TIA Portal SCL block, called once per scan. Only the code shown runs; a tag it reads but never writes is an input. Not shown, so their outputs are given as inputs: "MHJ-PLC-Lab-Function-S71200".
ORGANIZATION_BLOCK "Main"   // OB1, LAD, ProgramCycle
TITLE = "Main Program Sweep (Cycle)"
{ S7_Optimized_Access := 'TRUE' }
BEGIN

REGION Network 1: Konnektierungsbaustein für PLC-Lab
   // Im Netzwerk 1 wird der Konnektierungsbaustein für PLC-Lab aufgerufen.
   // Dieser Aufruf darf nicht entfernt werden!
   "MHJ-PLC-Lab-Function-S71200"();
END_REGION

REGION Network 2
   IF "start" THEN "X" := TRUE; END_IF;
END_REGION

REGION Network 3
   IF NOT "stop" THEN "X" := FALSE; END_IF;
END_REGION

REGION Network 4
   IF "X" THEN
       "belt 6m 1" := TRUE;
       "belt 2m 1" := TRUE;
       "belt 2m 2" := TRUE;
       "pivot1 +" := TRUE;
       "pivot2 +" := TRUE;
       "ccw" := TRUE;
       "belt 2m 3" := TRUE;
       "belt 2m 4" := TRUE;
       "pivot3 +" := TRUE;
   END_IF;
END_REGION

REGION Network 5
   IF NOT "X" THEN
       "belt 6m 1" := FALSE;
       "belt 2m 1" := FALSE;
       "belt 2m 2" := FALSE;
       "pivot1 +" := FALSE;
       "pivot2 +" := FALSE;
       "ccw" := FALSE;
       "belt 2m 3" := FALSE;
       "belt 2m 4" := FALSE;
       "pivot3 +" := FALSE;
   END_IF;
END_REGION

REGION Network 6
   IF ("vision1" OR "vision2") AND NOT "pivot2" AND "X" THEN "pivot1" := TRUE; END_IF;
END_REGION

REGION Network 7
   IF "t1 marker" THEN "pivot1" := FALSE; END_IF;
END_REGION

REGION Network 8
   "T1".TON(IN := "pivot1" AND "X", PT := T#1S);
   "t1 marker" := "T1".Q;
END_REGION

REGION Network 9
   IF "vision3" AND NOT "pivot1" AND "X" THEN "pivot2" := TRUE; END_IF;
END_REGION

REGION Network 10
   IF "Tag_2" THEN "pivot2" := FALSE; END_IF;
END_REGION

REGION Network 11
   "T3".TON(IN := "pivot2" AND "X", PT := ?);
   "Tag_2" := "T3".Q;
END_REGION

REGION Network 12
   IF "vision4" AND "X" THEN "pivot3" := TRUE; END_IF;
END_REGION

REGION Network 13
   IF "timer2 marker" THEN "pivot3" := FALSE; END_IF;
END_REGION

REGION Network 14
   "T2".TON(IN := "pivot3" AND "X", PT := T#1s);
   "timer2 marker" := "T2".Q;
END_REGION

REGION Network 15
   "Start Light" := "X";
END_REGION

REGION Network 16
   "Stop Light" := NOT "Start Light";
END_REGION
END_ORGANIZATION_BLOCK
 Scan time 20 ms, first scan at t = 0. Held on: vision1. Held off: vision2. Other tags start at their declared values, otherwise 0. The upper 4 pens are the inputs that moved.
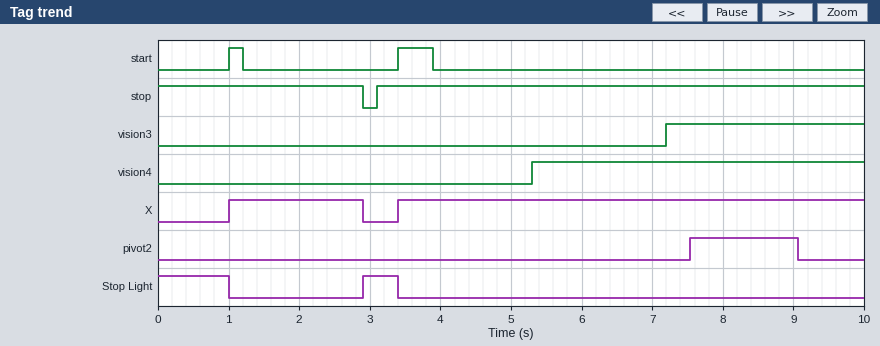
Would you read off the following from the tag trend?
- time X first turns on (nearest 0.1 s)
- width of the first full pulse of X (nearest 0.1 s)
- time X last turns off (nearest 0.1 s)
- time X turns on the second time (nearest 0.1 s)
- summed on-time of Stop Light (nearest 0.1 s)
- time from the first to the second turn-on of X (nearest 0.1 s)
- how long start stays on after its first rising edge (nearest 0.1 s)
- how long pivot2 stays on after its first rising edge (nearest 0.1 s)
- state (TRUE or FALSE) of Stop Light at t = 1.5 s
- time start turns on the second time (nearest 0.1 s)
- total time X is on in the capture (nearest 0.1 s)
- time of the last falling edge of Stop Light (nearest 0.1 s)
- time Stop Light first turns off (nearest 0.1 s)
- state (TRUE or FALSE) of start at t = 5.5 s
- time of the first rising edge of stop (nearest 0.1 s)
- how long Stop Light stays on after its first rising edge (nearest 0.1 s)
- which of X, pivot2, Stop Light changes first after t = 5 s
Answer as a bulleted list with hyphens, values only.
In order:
- 1.0 s
- 1.9 s
- 2.9 s
- 3.4 s
- 1.5 s
- 2.4 s
- 0.2 s
- 1.5 s
- FALSE
- 3.4 s
- 8.5 s
- 3.4 s
- 1.0 s
- FALSE
- 3.1 s
- 0.5 s
- pivot2
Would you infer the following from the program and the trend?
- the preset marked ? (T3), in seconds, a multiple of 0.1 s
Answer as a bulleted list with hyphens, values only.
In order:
- 1.5 s
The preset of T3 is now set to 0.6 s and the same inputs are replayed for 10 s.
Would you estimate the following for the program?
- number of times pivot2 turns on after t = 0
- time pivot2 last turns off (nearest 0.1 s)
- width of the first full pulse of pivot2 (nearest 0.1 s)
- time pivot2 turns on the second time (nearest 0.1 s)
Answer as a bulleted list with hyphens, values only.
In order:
- 2
- 9.8 s
- 0.6 s
- 9.2 s
